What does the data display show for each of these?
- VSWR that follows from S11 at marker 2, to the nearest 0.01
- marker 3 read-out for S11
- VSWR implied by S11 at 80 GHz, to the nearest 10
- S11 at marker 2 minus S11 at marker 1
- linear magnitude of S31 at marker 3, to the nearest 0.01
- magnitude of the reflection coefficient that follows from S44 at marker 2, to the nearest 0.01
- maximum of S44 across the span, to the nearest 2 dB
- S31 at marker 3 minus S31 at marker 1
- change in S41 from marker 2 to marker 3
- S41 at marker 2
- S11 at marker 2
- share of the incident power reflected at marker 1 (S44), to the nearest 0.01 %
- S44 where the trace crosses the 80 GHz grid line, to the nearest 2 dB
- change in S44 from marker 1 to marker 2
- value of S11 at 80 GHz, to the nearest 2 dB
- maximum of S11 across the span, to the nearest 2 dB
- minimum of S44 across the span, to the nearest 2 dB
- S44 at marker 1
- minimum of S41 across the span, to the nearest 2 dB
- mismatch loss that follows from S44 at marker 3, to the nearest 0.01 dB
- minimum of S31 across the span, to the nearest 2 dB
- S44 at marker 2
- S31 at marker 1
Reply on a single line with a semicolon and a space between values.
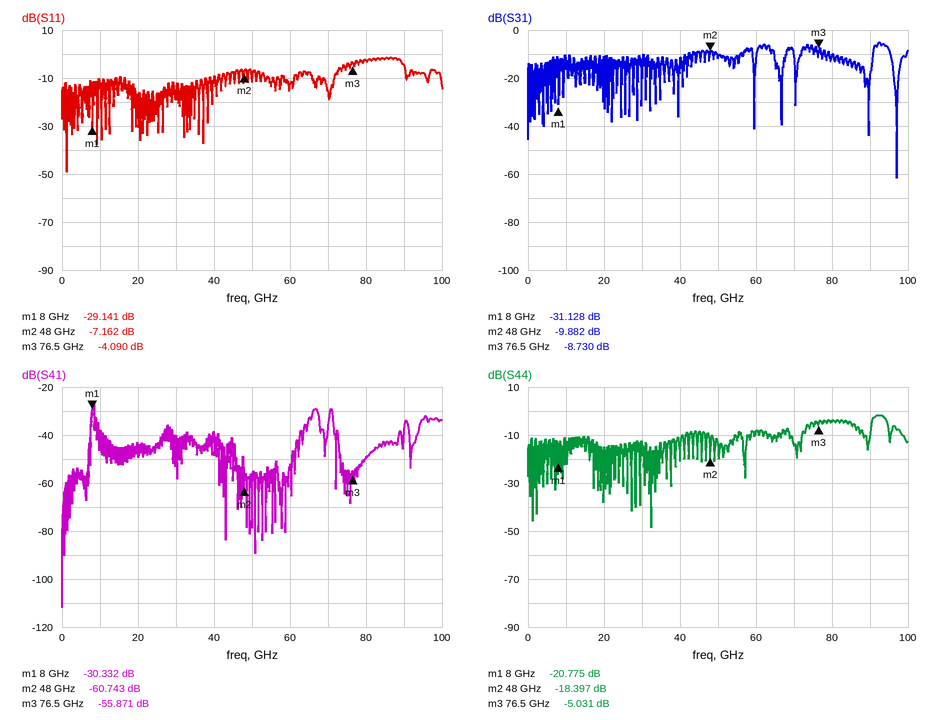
2.56; -4.090 dB; 10; 21.979 dB; 0.37; 0.12; -2 dB; 22.398 dB; 4.872 dB; -60.743 dB; -7.162 dB; 0.84 %; -4 dB; 2.378 dB; -2 dB; -2 dB; -48 dB; -20.775 dB; -112 dB; 1.64 dB; -62 dB; -18.397 dB; -31.128 dB
